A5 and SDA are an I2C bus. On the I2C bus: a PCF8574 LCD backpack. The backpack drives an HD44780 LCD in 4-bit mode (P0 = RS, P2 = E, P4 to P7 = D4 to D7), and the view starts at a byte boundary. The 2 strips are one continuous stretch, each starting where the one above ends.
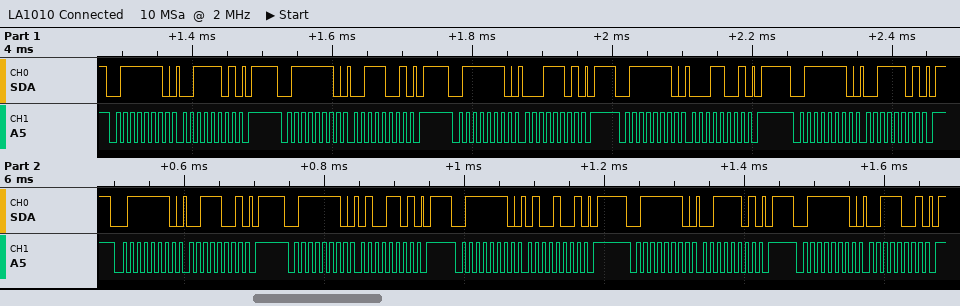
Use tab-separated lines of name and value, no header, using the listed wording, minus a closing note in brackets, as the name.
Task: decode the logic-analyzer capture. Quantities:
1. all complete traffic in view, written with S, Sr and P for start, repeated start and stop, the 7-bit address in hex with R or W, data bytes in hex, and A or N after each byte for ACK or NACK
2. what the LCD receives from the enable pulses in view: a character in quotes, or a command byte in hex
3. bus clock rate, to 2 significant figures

all complete traffic in view, written with S, Sr and P for start, repeated start and stop, the 7-bit address in hex with R or W, data bytes in hex, and A or N after each byte for ACK or NACK	S 3FW A 3D A P S 3FW A 39 A P S 3FW A 1D A P S 3FW A 19 A P S 3FW A 3D A P S 3FW A 39 A P S 3FW A 4D A P S 3FW A 49 A P S 3FW A 3D A P S 3FW A 39 A P
what the LCD receives from the enable pulses in view: a character in quotes, or a command byte in hex	'1' '4'
bus clock rate, to 2 significant figures	100 kHz
